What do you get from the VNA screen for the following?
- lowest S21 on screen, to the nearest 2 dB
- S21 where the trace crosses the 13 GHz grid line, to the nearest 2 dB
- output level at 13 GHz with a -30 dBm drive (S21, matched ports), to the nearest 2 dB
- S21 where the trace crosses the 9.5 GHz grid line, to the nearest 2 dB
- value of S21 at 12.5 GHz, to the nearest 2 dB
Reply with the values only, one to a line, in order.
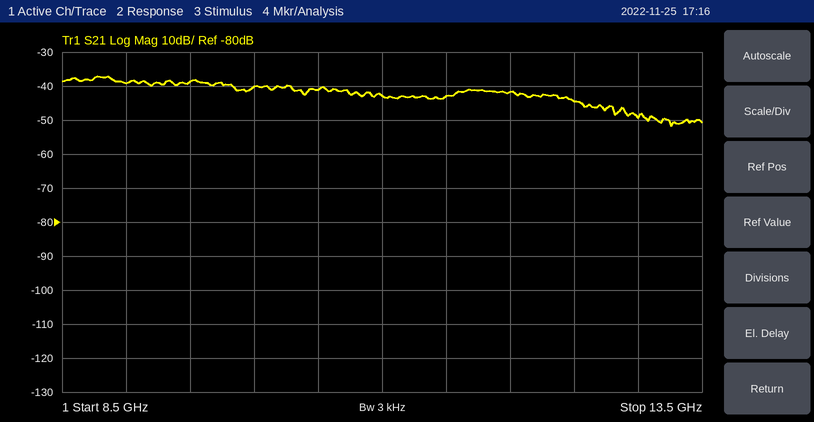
-52 dB
-50 dB
-80 dBm
-38 dB
-44 dB
